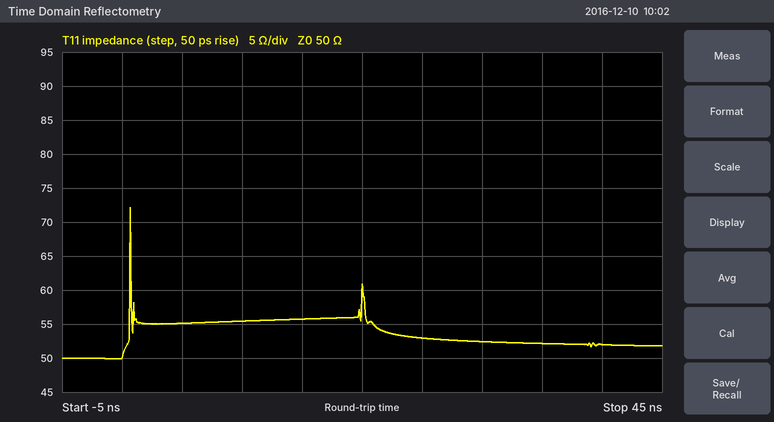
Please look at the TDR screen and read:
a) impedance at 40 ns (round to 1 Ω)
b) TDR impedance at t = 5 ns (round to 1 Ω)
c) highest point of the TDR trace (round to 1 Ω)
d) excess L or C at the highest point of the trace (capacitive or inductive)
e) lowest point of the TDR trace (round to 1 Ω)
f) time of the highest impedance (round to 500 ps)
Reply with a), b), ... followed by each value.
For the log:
a) 52 Ω
b) 55 Ω
c) 72 Ω
d) inductive
e) 50 Ω
f) 500 ps
